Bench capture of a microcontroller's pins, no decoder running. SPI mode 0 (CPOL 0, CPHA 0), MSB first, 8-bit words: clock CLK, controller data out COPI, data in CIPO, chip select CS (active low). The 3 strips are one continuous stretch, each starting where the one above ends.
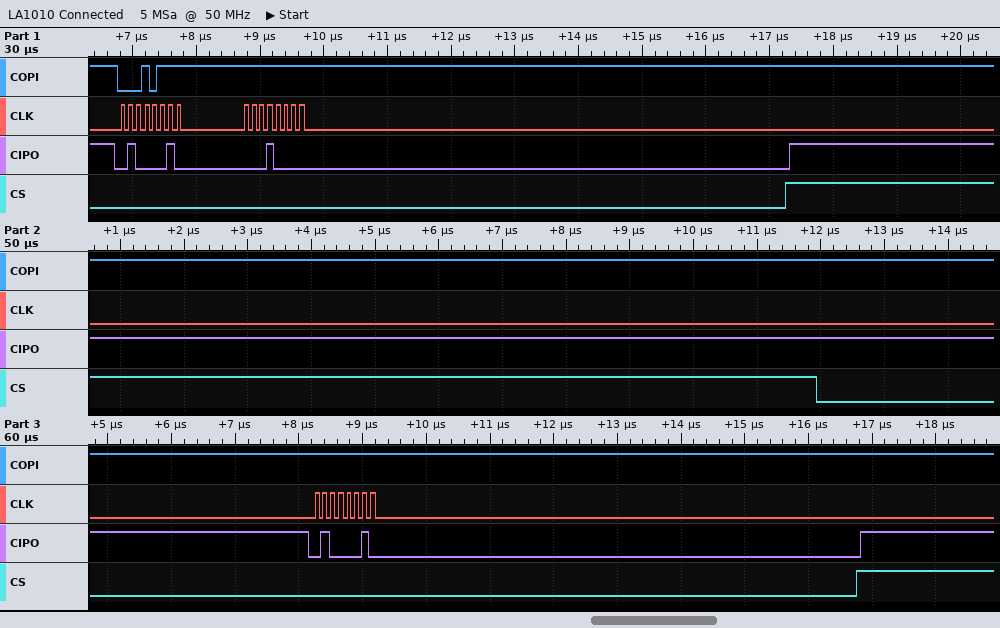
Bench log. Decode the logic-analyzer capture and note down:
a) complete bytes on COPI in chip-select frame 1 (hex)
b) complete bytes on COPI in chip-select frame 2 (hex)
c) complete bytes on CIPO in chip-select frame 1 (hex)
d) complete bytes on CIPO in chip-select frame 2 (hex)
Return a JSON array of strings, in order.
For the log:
["17 FF", "FF", "42 10", "42"]
